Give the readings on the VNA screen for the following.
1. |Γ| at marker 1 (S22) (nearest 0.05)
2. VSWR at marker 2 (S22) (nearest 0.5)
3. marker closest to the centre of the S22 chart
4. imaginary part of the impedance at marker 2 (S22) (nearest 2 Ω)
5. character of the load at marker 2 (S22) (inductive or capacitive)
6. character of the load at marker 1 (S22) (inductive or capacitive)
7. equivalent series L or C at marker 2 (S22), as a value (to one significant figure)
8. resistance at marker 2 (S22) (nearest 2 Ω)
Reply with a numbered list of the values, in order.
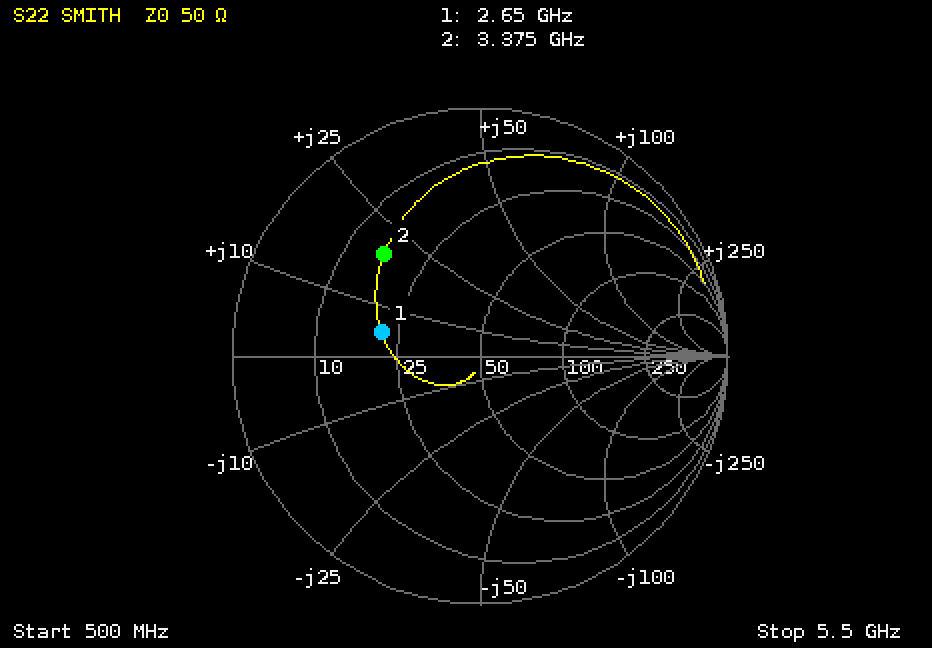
1. 0.40
2. 3.5
3. marker 1
4. +20 Ω
5. inductive
6. inductive
7. 900 pH
8. 16 Ω
